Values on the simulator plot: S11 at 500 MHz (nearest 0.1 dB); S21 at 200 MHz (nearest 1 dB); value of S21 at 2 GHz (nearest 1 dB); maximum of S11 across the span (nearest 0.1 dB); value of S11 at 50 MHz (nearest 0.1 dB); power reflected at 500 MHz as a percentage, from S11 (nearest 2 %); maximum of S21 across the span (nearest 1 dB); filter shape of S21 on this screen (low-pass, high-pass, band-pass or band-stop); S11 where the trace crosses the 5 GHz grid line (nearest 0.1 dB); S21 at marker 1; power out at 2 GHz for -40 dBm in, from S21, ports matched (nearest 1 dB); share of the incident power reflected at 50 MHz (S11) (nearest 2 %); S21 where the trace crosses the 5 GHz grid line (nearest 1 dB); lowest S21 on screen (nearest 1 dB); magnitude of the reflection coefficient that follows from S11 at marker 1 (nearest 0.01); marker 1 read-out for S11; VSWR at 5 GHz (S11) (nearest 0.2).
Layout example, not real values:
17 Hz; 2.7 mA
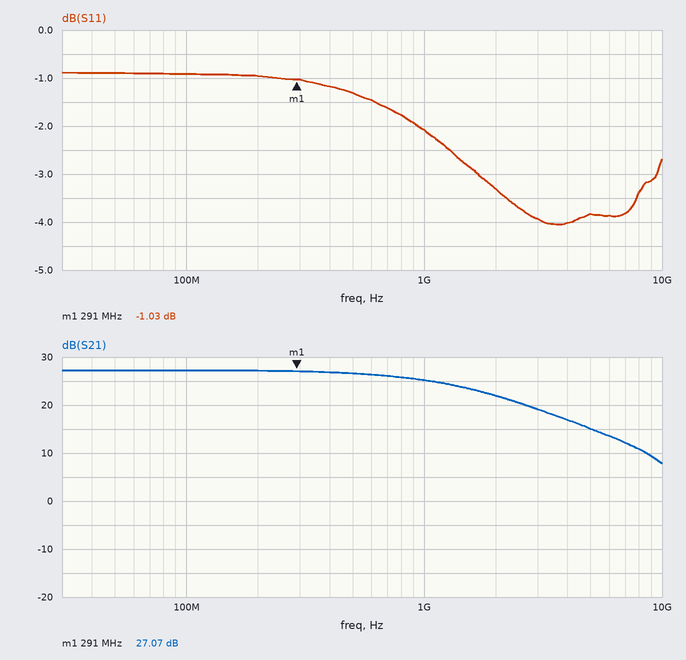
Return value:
-1.3 dB; 27 dB; 22 dB; -0.9 dB; -0.9 dB; 74 %; 27 dB; low-pass; -3.8 dB; 27.07 dB; -18 dBm; 82 %; 15 dB; 8 dB; 0.89; -1.03 dB; 4.6
